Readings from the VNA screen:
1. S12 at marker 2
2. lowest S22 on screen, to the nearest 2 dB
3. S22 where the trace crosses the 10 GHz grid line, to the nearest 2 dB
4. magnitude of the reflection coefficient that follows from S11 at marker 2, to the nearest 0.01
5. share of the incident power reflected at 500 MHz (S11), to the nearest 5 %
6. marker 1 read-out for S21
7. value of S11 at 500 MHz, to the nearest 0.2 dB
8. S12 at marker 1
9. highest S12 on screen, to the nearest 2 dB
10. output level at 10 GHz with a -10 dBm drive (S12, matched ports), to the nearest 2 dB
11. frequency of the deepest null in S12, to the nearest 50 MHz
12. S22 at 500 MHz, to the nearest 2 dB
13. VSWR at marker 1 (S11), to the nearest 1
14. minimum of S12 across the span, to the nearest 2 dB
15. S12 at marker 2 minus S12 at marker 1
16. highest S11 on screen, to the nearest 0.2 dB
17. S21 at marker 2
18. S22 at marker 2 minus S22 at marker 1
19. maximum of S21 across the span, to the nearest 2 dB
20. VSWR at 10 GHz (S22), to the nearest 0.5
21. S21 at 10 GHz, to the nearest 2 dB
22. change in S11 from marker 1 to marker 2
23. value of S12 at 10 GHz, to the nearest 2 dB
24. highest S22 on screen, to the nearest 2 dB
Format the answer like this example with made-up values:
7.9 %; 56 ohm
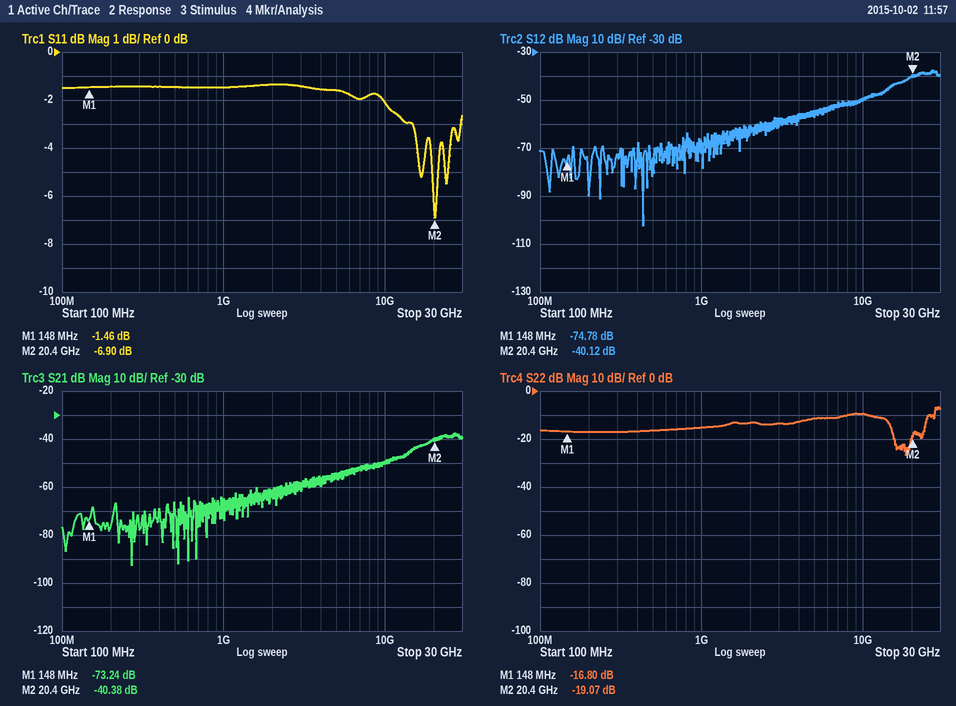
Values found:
-40.12 dB; -26 dB; -10 dB; 0.45; 70 %; -73.24 dB; -1.4 dB; -74.78 dB; -38 dB; -60 dBm; 450 MHz; -16 dB; 12; -102 dB; 34.66 dB; -1.4 dB; -40.38 dB; -2.27 dB; -38 dB; 2.0; -50 dB; -5.44 dB; -50 dB; -6 dB
